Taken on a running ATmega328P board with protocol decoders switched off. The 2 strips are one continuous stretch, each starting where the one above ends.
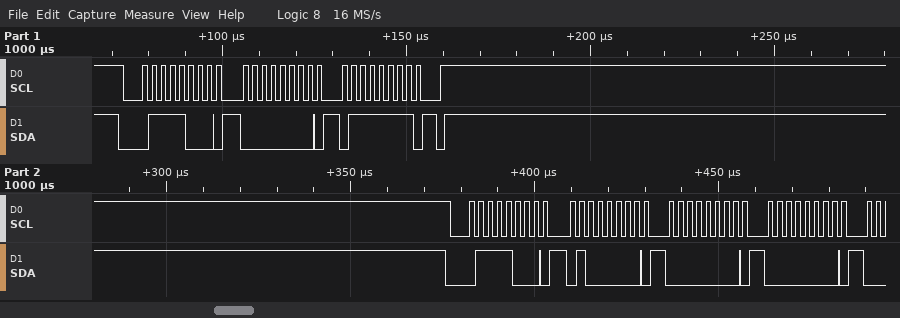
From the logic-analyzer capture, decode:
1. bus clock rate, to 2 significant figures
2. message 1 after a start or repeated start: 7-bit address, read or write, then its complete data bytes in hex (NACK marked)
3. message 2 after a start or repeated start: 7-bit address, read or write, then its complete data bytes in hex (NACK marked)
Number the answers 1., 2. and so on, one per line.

1. 400 kHz
2. 0x3C write: 00 7F
3. 0x3C write: 40 00 00
